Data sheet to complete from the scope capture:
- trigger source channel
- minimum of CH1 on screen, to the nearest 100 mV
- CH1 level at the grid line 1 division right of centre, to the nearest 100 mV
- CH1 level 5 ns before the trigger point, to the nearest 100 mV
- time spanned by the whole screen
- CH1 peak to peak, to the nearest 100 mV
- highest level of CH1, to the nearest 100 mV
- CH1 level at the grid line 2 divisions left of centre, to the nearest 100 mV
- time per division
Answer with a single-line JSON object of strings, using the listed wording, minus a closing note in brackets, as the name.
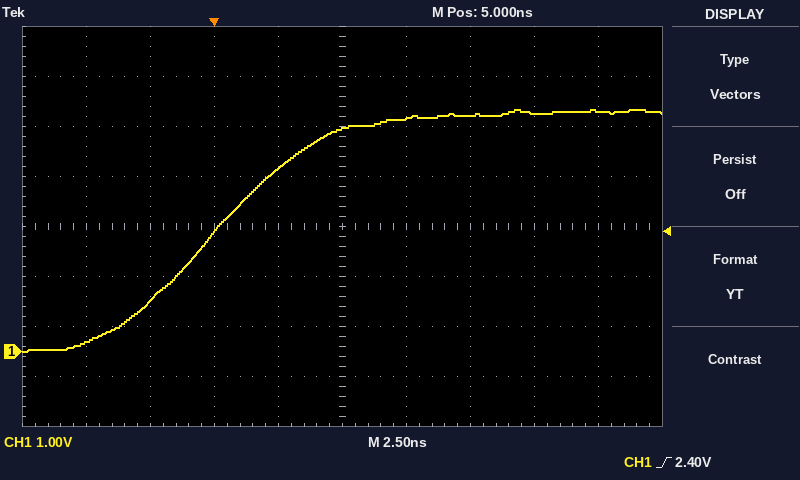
{"trigger source channel": "CH1", "minimum of CH1 on screen, to the nearest 100 mV": "0.0 V", "CH1 level at the grid line 1 division right of centre, to the nearest 100 mV": "4.7 V", "CH1 level 5 ns before the trigger point, to the nearest 100 mV": "200 mV", "time spanned by the whole screen": "25 ns", "CH1 peak to peak, to the nearest 100 mV": "4.8 V", "highest level of CH1, to the nearest 100 mV": "4.8 V", "CH1 level at the grid line 2 divisions left of centre, to the nearest 100 mV": "2.4 V", "time per division": "2.5 ns"}
